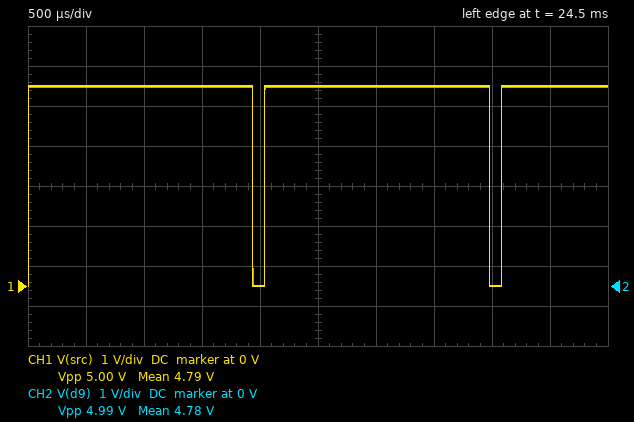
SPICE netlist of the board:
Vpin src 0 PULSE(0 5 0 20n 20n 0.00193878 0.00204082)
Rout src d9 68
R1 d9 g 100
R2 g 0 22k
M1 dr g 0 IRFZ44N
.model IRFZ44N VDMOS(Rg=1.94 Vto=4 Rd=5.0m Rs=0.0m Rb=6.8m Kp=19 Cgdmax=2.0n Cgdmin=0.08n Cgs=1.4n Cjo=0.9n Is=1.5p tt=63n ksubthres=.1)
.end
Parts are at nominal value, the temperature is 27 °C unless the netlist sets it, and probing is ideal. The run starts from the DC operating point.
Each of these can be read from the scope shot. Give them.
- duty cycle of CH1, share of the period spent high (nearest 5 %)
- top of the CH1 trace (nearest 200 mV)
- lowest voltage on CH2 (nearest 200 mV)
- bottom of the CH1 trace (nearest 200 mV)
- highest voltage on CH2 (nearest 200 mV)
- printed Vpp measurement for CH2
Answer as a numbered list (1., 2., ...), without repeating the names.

1. 95 %
2. 5.0 V
3. 0 V
4. 0 V
5. 5.0 V
6. 4.99 V
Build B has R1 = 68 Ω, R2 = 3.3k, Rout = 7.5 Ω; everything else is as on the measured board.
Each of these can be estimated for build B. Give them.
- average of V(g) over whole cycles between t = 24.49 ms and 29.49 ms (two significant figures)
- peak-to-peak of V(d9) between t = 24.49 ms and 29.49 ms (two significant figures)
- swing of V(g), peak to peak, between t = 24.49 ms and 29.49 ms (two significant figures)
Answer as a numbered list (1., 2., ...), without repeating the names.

1. 4.6 V
2. 5.0 V
3. 4.9 V
